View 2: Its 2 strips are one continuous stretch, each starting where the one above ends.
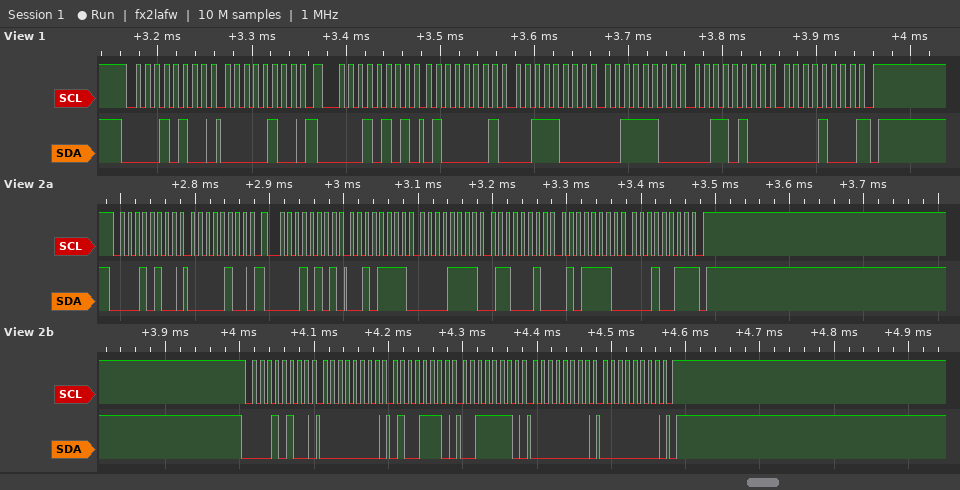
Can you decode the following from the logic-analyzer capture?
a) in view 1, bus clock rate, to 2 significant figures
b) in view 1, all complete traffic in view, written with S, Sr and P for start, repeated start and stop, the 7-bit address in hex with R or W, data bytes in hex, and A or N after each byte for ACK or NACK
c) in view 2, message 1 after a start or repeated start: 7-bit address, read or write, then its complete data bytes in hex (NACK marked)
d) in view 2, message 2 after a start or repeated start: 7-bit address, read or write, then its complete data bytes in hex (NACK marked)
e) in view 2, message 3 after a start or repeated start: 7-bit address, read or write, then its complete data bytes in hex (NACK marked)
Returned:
100 kHz
S 0AW A 04 A Sr 0AR A 41 A 38 A 3C A 34 A 08 N P
0x0A write: 04
0x0A read: 2F 0F 62 5E 13 NACK
0x0A write: 00 4E 3E 00 00
